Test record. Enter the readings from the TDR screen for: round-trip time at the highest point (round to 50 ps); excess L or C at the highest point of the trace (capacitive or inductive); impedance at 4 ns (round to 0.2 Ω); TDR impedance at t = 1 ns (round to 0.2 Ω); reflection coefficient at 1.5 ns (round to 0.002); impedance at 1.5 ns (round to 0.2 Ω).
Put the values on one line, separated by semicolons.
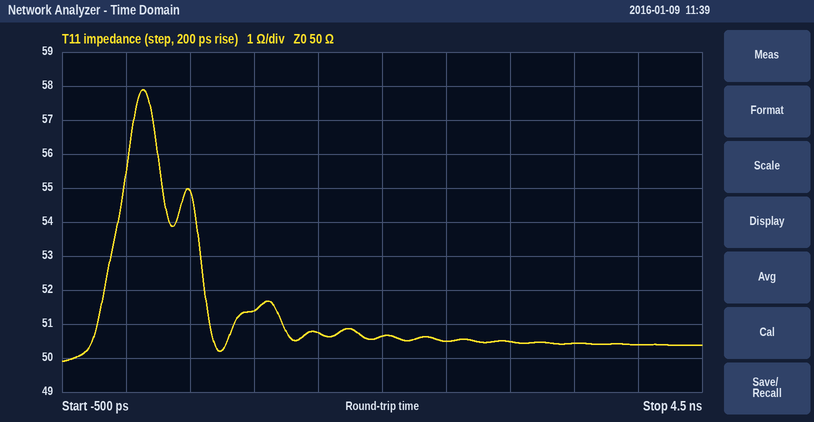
150 ps; inductive; 50.4 Ω; 51.4 Ω; +0.008; 50.8 Ω
